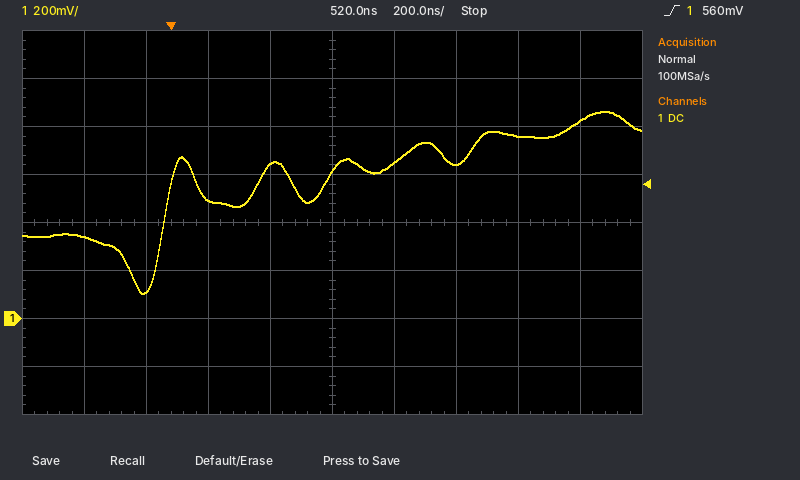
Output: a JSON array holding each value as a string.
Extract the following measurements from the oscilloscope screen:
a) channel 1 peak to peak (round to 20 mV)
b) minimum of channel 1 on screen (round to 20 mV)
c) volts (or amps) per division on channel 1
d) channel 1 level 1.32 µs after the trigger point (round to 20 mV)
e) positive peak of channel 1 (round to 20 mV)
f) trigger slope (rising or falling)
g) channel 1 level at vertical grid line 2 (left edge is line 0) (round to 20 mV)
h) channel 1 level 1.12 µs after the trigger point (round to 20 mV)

["760 mV", "100 mV", "200 mV", "820 mV", "860 mV", "rising", "120 mV", "760 mV"]
